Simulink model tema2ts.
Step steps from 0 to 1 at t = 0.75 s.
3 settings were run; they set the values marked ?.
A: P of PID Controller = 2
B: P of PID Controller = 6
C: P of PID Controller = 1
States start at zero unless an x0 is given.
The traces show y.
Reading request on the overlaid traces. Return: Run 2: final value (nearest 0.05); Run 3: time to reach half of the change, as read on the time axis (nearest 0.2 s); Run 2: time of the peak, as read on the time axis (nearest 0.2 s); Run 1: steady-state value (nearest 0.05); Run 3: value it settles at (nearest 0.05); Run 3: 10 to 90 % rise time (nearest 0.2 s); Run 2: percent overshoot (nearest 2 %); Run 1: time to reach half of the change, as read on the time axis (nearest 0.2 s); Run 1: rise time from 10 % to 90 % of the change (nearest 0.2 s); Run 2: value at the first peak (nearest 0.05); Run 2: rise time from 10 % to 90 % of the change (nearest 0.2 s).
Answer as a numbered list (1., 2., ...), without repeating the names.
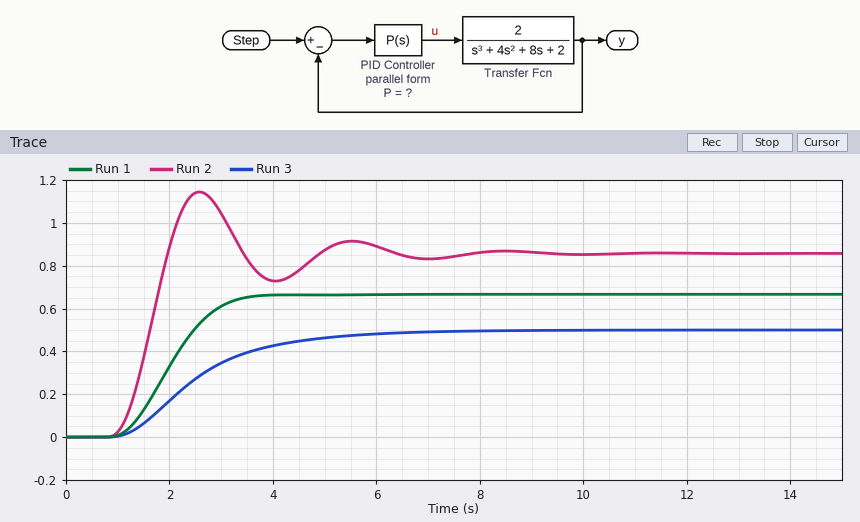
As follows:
1. 0.85
2. 2.4 s
3. 2.6 s
4. 0.65
5. 0.50
6. 3.2 s
7. 34 %
8. 2.0 s
9. 1.6 s
10. 1.15
11. 0.8 s
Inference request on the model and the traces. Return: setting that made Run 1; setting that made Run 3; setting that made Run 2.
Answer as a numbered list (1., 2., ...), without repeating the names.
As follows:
1. A
2. C
3. B
